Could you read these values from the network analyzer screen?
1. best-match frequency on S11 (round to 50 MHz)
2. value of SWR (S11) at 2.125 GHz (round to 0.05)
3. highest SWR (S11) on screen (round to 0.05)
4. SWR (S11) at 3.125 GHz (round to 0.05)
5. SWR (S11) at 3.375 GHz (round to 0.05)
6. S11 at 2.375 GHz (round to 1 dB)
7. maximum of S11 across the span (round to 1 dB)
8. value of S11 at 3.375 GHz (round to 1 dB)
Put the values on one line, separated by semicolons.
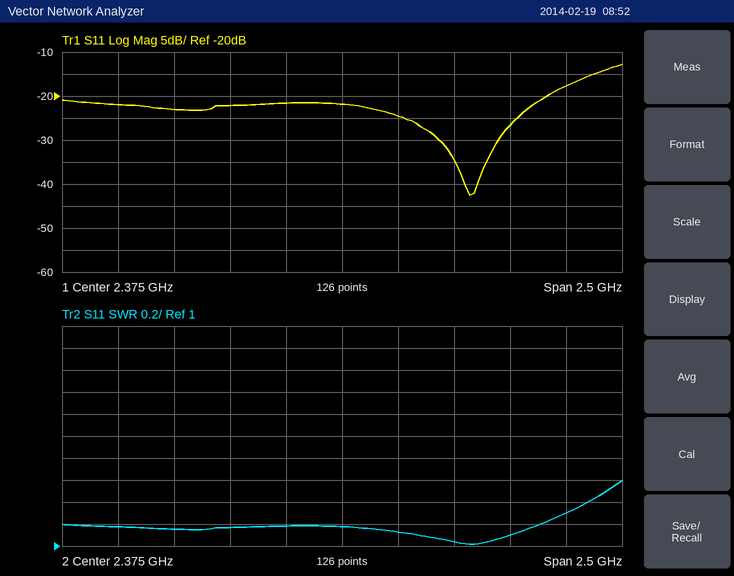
2.95 GHz; 1.20; 1.60; 1.10; 1.30; -22 dB; -13 dB; -18 dB
